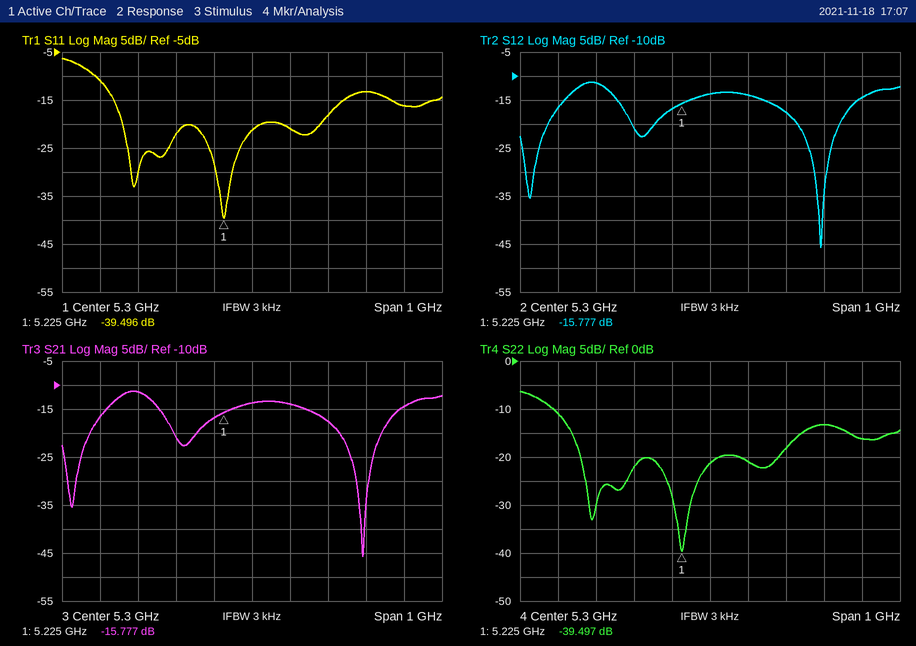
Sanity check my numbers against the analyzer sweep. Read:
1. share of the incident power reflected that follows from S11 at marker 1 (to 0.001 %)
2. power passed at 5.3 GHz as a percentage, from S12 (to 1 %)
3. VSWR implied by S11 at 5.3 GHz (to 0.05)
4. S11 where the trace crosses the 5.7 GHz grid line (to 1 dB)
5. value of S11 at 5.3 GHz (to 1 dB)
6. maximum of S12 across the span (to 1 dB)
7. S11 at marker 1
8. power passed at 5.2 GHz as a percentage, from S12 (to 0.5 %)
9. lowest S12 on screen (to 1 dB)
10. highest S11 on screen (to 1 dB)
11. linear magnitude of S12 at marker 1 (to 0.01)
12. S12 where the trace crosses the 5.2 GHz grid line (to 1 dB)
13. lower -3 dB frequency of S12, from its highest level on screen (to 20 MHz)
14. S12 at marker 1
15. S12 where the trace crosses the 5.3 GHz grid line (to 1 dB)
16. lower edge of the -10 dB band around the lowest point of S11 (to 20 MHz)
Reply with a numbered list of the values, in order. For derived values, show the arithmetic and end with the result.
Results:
1. 10^(-39.496/10) ≈ 0.011 %
2. 10^(-14/10) ≈ 4 %
3. |Γ| = 10^(-21/20) = 0.0891; VSWR = (1 + 0.0891)/(1 − 0.0891) ≈ 1.20
4. -16 dB
5. -21 dB
6. -11 dB
7. -39.496 dB
8. 10^(-17/10) ≈ 2.0 %
9. -46 dB
10. -6 dB
11. 10^(-15.777/20) ≈ 0.16
12. -17 dB
13. 4.92 GHz
14. -15.777 dB
15. -14 dB
16. 4.88 GHz
